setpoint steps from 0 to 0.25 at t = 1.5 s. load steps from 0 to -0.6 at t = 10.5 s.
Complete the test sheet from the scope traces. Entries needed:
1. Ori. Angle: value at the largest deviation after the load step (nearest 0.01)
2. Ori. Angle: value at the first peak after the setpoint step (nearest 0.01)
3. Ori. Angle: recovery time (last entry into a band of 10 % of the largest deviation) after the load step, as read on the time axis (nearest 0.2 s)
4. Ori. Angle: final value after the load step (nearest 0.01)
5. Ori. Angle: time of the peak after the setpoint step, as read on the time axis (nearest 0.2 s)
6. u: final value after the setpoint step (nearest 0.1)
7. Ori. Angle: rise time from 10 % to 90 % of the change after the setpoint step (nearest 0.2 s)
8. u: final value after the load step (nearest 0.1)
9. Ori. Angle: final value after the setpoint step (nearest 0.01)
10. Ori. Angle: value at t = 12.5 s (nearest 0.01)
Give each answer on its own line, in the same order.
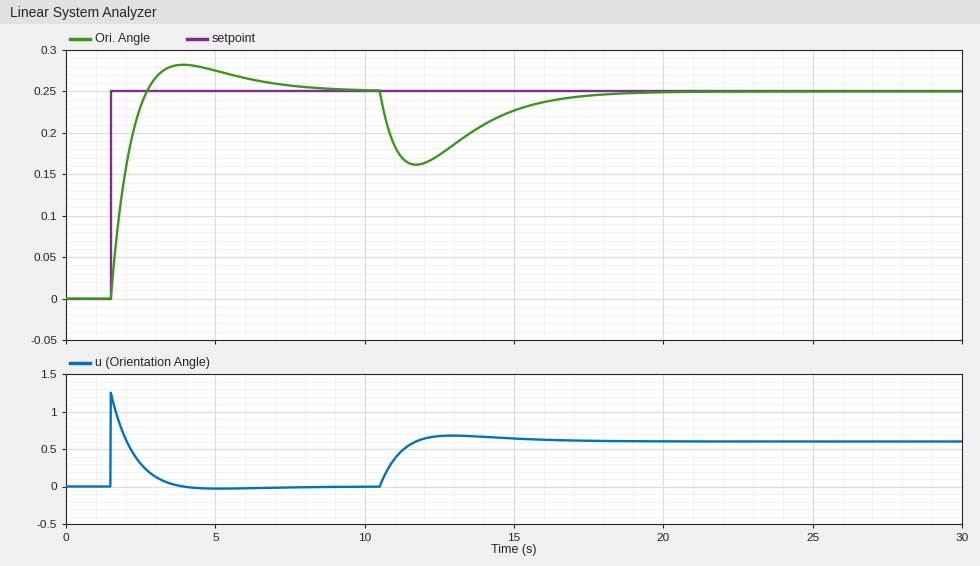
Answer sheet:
0.16
0.28
16.6 s
0.25
4.0 s
0.0
0.8 s
0.6
0.25
0.17
